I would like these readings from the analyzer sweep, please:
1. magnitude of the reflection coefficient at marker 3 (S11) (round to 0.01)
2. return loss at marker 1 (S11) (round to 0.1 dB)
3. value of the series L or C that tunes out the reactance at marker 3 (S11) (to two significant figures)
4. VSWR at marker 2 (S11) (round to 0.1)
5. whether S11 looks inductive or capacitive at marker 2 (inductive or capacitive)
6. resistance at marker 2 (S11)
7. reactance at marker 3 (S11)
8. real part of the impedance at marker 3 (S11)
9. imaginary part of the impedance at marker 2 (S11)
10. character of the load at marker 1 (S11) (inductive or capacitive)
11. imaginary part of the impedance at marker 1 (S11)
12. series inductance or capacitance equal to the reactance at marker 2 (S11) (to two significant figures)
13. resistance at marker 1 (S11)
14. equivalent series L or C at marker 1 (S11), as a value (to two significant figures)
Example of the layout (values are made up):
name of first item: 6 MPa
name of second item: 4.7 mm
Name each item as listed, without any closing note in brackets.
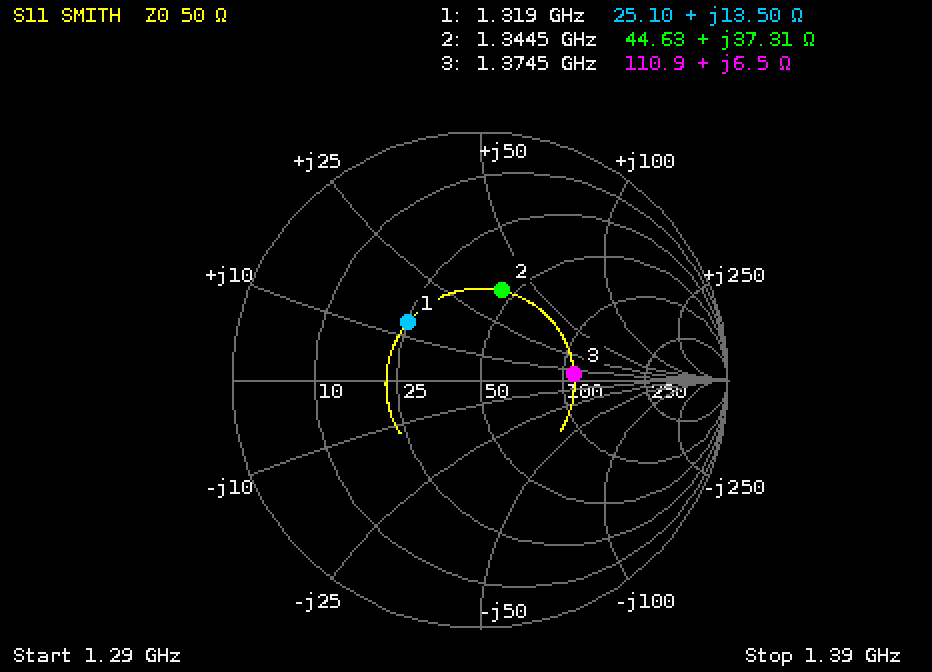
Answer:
magnitude of the reflection coefficient at marker 3 (S11): 0.38
return loss at marker 1 (S11): 8.6 dB
value of the series L or C that tunes out the reactance at marker 3 (S11): 18 pF
VSWR at marker 2 (S11): 2.2
whether S11 looks inductive or capacitive at marker 2: inductive
resistance at marker 2: 44.63 Ω
reactance at marker 3: +6.5 Ω
real part of the impedance at marker 3: 110.9 Ω
imaginary part of the impedance at marker 2: +37.31 Ω
character of the load at marker 1 (S11): inductive
imaginary part of the impedance at marker 1: +13.50 Ω
series inductance or capacitance equal to the reactance at marker 2 (S11): 4.4 nH
resistance at marker 1: 25.10 Ω
equivalent series L or C at marker 1 (S11), as a value: 1.6 nH
